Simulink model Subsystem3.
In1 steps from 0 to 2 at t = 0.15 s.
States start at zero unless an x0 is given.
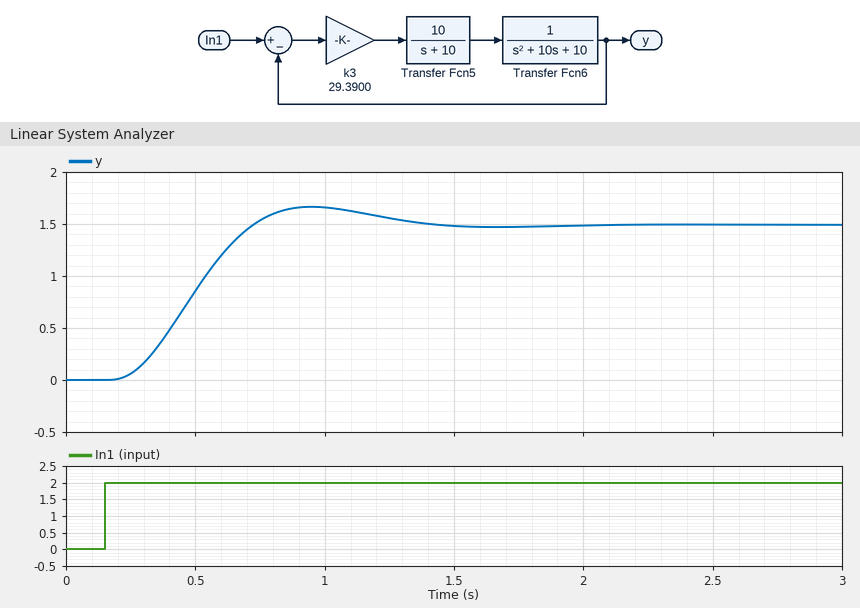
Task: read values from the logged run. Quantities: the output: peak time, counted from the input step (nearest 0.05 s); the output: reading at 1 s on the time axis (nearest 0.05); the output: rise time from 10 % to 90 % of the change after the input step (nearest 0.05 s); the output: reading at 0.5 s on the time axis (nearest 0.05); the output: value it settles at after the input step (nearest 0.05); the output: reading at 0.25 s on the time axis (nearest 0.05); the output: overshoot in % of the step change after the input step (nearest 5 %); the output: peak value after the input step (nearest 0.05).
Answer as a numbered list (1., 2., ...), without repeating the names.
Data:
1. 0.80 s
2. 1.65
3. 0.35 s
4. 0.85
5. 1.50
6. 0.05
7. 10 %
8. 1.65
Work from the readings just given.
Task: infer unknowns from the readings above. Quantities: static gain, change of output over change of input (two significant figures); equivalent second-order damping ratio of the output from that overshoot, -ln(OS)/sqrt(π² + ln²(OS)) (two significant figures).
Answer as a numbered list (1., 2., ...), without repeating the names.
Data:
1. 0.75
2. 0.59
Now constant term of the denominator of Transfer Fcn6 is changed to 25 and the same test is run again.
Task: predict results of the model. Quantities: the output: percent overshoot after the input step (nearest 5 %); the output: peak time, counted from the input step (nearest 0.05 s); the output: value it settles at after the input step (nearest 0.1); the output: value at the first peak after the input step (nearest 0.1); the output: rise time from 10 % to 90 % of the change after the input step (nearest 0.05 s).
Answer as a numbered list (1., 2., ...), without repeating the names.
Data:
1. 15 %
2. 0.65 s
3. 1.1
4. 1.2
5. 0.30 s
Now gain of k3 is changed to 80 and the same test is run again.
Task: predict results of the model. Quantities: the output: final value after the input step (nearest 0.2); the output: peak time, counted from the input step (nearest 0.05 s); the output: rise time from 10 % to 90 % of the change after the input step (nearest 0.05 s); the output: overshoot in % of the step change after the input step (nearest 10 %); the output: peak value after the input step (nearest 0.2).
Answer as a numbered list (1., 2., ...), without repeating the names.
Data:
1. 1.8
2. 0.50 s
3. 0.20 s
4. 40 %
5. 2.6
